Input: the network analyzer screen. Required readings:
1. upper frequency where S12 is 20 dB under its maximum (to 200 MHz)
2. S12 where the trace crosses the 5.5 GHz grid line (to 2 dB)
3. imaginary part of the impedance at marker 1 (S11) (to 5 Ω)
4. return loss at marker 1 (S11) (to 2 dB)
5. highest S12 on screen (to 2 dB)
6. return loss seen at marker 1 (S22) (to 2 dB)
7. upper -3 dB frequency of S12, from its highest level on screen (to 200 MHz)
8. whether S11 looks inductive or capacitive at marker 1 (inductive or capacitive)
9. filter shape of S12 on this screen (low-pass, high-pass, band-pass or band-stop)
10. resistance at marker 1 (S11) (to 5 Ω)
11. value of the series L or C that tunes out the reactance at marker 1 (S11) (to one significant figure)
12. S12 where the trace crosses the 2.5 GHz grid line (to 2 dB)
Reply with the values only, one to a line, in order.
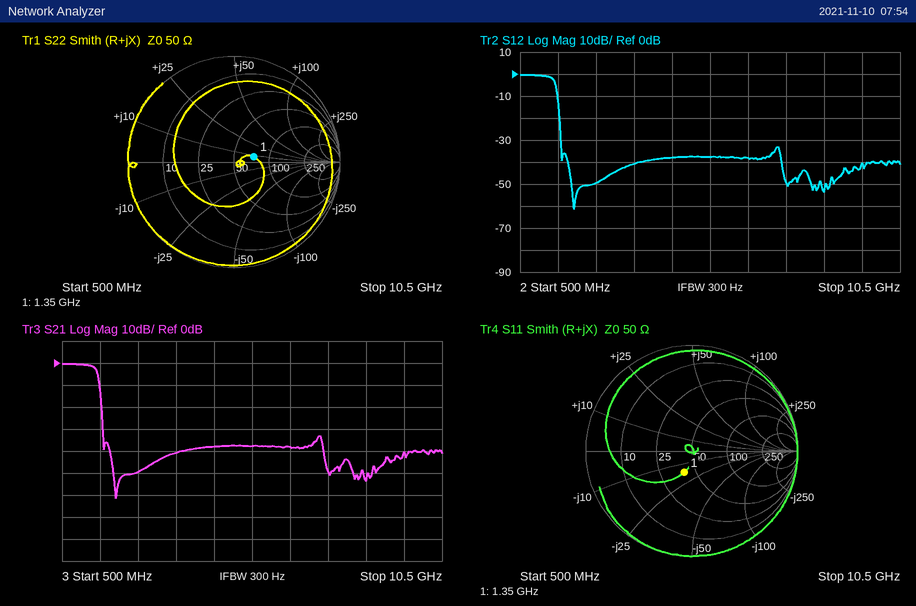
1.6 GHz
-38 dB
-15 Ω
14 dB
0 dB
14 dB
1.4 GHz
capacitive
low-pass
40 Ω
2 nH
-50 dB
